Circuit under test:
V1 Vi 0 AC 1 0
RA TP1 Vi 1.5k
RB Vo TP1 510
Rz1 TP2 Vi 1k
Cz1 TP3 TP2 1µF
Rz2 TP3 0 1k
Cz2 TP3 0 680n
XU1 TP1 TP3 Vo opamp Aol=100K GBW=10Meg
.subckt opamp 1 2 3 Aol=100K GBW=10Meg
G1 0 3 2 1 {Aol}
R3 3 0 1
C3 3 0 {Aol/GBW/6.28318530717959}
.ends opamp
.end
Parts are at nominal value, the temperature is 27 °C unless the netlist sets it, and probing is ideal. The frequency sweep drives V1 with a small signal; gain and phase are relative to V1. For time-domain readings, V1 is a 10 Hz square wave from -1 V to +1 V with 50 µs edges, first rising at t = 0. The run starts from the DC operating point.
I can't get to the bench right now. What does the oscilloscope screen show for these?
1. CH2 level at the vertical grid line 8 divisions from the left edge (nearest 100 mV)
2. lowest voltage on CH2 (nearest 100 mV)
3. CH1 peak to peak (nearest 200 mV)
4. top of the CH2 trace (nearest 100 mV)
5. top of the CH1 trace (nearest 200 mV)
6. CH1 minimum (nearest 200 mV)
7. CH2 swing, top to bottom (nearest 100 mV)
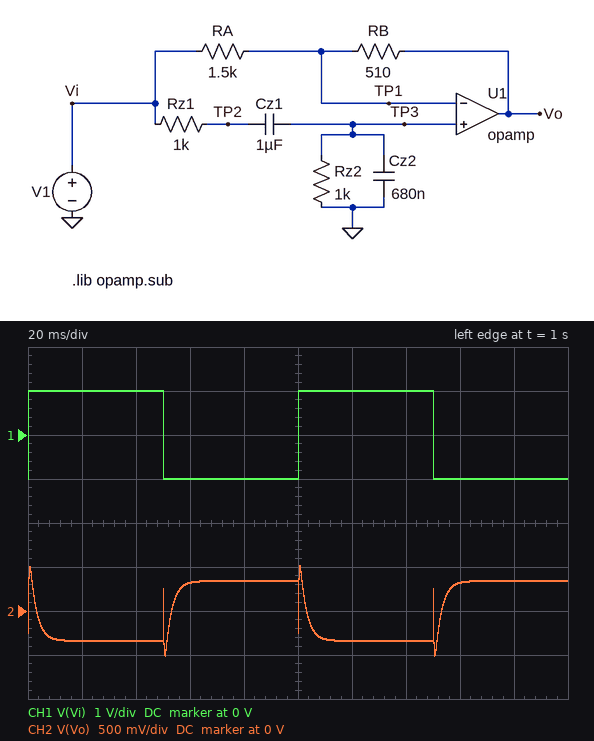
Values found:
300 mV
-500 mV
2.0 V
500 mV
1.0 V
-1.0 V
1.0 V
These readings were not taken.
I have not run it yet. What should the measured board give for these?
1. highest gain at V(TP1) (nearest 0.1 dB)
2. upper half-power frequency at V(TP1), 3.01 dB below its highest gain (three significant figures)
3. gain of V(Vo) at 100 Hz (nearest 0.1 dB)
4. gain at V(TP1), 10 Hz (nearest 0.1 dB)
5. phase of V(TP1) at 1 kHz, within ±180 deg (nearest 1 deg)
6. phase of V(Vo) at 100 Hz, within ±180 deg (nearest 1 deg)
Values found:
-8.6 dB
682 Hz
-14.0 dB
-24.1 dB
-57 deg
66 deg
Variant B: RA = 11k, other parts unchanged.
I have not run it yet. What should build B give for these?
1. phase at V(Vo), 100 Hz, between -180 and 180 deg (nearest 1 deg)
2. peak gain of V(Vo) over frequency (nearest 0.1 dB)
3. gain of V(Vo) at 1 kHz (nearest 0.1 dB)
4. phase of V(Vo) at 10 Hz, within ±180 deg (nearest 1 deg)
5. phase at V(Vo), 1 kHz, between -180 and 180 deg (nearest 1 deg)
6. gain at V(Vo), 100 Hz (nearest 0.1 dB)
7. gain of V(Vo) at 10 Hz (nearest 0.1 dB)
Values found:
27 deg
-9.3 dB
-14.3 dB
119 deg
-69 deg
-10.0 dB
-22.7 dB
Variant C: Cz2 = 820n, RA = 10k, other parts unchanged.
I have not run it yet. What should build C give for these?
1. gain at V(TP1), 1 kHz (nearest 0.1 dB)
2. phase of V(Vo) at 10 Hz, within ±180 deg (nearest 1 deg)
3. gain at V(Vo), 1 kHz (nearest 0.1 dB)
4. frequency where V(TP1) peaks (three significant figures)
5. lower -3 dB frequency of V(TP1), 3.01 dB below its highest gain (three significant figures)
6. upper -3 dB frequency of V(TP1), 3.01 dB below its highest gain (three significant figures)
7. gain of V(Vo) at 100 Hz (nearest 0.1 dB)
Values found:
-15.2 dB
122 deg
-15.7 dB
176 Hz
51.6 Hz
599 Hz
-10.4 dB
